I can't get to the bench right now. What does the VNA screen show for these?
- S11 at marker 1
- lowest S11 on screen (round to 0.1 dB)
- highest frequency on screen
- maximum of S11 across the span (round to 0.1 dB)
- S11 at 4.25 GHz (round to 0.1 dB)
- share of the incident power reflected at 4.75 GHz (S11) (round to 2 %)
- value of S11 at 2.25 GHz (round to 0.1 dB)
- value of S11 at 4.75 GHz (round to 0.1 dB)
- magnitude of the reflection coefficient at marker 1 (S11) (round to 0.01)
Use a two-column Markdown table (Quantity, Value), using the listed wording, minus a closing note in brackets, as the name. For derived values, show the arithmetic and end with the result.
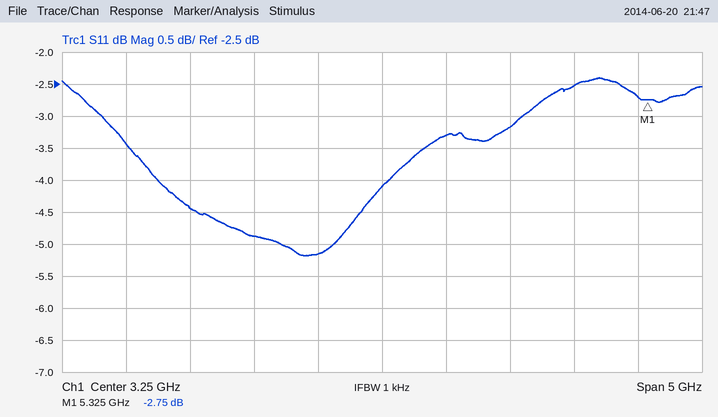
| Quantity | Value |
|---|---|
| S11 at marker 1 | -2.75 dB |
| lowest S11 on screen | -5.2 dB |
| highest frequency on screen | 5.75 GHz |
| maximum of S11 across the span | -2.4 dB |
| S11 at 4.25 GHz | -3.2 dB |
| share of the incident power reflected at 4.75 GHz (S11) | 10^(-2.5/10) ≈ 56 % |
| value of S11 at 2.25 GHz | -4.9 dB |
| value of S11 at 4.75 GHz | -2.5 dB |
| magnitude of the reflection coefficient at marker 1 (S11) | 10^(-2.75/20) ≈ 0.73 |
